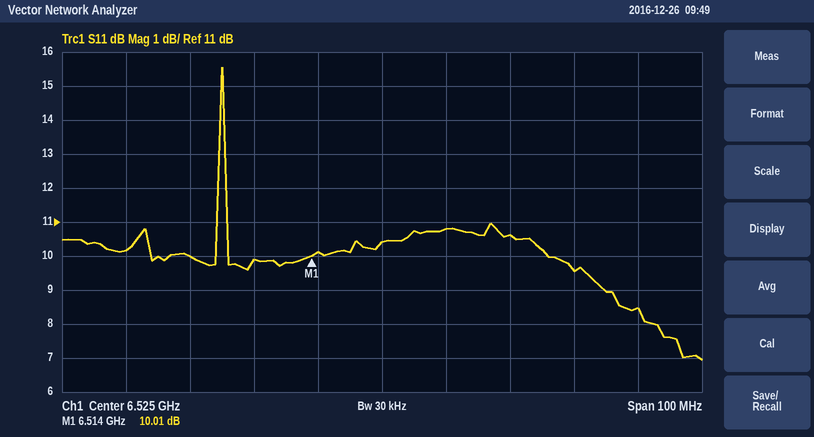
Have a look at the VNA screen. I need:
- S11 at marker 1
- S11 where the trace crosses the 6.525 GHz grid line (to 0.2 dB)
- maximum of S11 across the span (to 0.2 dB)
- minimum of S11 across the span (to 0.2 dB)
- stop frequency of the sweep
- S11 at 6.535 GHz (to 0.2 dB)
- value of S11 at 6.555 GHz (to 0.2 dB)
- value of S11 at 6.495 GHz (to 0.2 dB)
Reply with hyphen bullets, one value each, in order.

- 10.01 dB
- 10.4 dB
- 15.6 dB
- 7.0 dB
- 6.575 GHz
- 10.8 dB
- 9.6 dB
- 10.0 dB
